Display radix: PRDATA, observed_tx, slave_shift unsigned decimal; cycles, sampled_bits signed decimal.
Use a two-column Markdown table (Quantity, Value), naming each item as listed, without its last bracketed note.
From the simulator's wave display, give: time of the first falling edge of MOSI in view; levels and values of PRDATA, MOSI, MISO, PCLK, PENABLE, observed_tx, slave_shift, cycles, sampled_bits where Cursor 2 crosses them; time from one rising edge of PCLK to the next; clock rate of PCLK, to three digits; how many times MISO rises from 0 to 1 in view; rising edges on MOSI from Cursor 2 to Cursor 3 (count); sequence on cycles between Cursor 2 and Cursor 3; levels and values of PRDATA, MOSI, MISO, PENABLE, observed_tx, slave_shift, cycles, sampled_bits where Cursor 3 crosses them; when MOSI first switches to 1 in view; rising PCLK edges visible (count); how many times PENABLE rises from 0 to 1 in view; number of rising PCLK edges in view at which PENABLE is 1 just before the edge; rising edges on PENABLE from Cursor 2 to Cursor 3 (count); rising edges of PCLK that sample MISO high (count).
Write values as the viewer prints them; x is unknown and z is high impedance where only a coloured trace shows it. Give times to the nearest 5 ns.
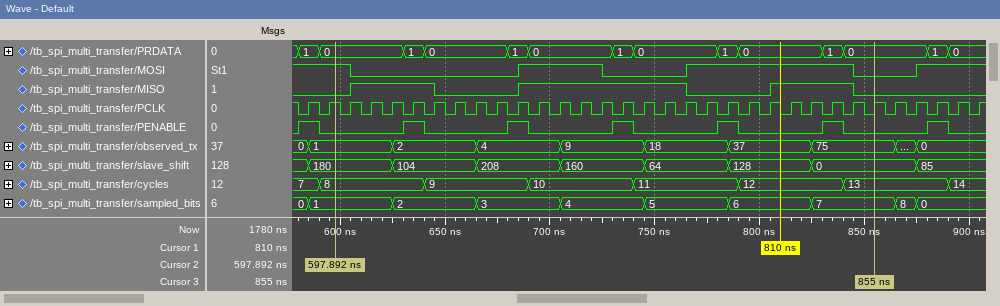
| Quantity | Value |
|---|---|
| time of the first falling edge of MOSI in view | 605 ns |
| levels and values of PRDATA, MOSI, MISO, PCLK, PENABLE, observed_tx, slave_shift, cycles, sampled_bits where Cursor 2 crosses them | PRDATA=0, MOSI=1, MISO=0, PCLK=1, PENABLE=0, observed_tx=1, slave_shift=180, cycles=8, sampled_bits=1 |
| time from one rising edge of PCLK to the next | 10 ns |
| clock rate of PCLK, to three digits | 100 MHz |
| how many times MISO rises from 0 to 1 in view | 3 |
| rising edges on MOSI from Cursor 2 to Cursor 3 | 2 |
| sequence on cycles between Cursor 2 and Cursor 3 | 8, 9, 10, 11, 12, 13 |
| levels and values of PRDATA, MOSI, MISO, PENABLE, observed_tx, slave_shift, cycles, sampled_bits where Cursor 3 crosses them | PRDATA=0, MOSI=0, MISO=0, PENABLE=0, observed_tx=75, slave_shift=0, cycles=13, sampled_bits=7 |
| when MOSI first switches to 1 in view | 685 ns |
| rising PCLK edges visible | 33 |
| how many times PENABLE rises from 0 to 1 in view | 7 |
| number of rising PCLK edges in view at which PENABLE is 1 just before the edge | 7 |
| rising edges on PENABLE from Cursor 2 to Cursor 3 | 5 |
| rising edges of PCLK that sample MISO high | 16 |
